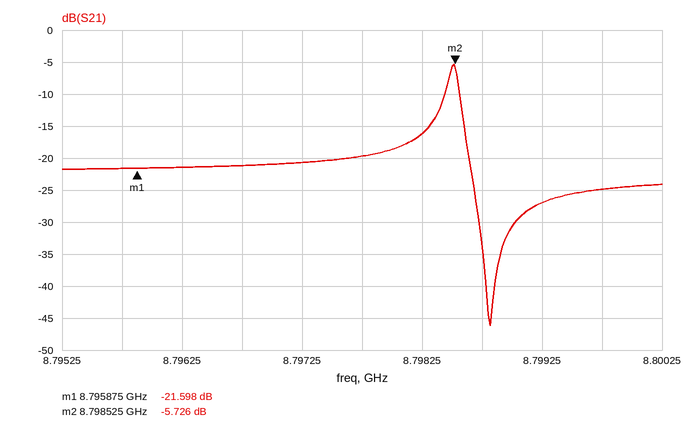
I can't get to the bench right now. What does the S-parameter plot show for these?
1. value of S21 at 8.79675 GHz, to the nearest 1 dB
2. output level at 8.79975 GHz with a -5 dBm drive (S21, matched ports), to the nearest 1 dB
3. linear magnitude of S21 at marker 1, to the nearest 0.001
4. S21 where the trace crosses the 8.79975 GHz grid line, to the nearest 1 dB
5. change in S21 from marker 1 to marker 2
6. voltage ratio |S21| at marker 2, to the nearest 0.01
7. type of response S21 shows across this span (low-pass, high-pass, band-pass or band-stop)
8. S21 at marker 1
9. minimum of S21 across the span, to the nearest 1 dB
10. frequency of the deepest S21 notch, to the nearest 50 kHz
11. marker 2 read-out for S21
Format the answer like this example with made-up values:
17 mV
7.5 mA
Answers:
-21 dB
-30 dBm
0.083
-25 dB
15.872 dB
0.52
band-pass
-21.598 dB
-46 dB
8.79880 GHz
-5.726 dB
